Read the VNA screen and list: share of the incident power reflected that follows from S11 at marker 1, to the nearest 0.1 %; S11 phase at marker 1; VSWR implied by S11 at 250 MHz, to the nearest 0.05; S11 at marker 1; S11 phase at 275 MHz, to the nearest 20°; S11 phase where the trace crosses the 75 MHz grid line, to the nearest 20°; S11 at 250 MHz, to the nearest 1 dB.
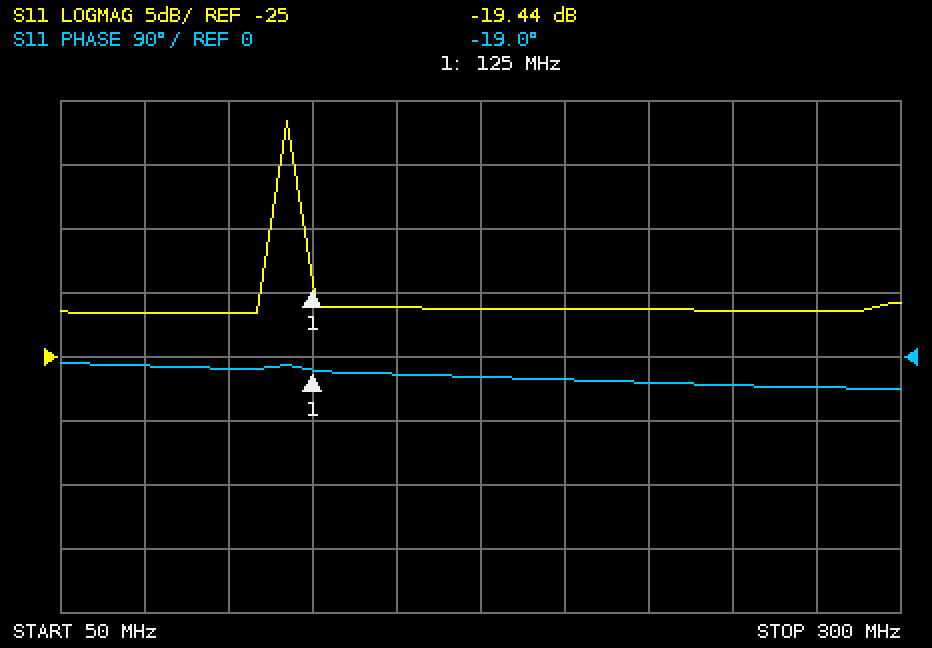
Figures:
1.1 %
-19.0°
1.20
-19.44 dB
-40°
-20°
-21 dB
